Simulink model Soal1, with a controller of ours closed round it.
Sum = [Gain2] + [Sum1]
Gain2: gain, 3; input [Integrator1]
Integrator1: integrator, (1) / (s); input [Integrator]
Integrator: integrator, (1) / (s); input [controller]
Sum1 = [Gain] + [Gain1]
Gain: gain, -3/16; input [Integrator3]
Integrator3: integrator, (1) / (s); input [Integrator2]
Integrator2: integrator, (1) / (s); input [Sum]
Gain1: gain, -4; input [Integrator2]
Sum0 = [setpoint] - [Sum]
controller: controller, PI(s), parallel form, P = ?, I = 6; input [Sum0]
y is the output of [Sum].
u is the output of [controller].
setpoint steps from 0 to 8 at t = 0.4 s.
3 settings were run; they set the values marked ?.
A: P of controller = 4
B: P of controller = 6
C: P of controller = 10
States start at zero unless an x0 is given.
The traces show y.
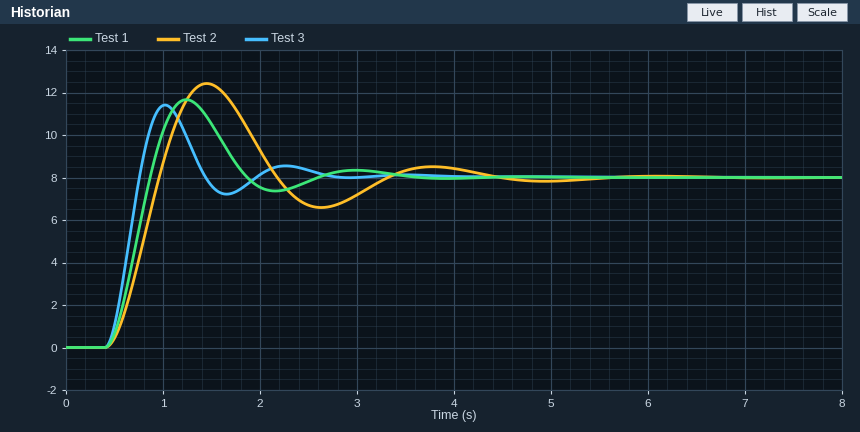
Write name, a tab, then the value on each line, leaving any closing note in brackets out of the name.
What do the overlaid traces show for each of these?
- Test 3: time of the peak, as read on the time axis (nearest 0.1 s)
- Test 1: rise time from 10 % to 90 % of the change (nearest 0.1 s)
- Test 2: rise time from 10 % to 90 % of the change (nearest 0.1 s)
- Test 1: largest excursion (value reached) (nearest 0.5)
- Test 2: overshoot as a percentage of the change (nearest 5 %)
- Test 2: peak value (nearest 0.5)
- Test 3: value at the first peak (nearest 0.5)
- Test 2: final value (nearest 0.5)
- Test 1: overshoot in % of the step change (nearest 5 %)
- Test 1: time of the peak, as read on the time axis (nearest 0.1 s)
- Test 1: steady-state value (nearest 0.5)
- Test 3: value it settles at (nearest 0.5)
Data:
Test 3: time of the peak, as read on the time axis	1.0 s
Test 1: rise time from 10 % to 90 % of the change	0.3 s
Test 2: rise time from 10 % to 90 % of the change	0.4 s
Test 1: largest excursion (value reached)	11.5
Test 2: overshoot as a percentage of the change	55 %
Test 2: peak value	12.5
Test 3: value at the first peak	11.5
Test 2: final value	8.0
Test 1: overshoot in % of the step change	45 %
Test 1: time of the peak, as read on the time axis	1.2 s
Test 1: steady-state value	8.0
Test 3: value it settles at	8.0
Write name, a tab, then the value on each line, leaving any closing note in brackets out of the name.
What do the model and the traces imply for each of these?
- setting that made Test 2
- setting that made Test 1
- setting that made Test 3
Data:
setting that made Test 2	A
setting that made Test 1	B
setting that made Test 3	C
